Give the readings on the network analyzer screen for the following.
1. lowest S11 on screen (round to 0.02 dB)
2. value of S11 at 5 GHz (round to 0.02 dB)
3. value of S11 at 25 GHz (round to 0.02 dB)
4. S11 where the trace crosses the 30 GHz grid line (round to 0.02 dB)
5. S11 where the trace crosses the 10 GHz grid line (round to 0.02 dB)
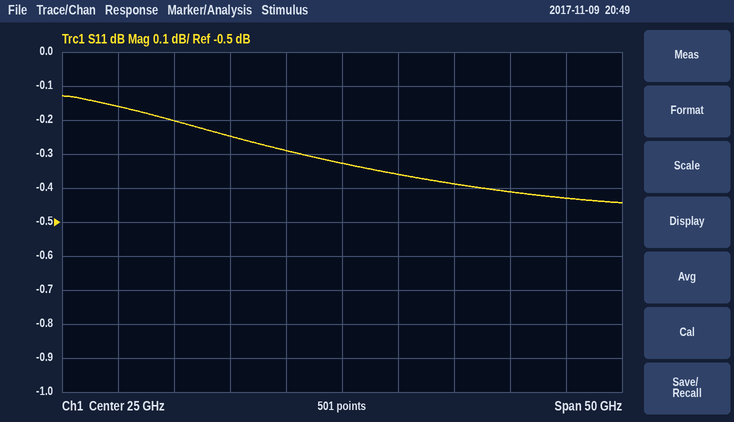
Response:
-0.44 dB
-0.16 dB
-0.32 dB
-0.36 dB
-0.20 dB
